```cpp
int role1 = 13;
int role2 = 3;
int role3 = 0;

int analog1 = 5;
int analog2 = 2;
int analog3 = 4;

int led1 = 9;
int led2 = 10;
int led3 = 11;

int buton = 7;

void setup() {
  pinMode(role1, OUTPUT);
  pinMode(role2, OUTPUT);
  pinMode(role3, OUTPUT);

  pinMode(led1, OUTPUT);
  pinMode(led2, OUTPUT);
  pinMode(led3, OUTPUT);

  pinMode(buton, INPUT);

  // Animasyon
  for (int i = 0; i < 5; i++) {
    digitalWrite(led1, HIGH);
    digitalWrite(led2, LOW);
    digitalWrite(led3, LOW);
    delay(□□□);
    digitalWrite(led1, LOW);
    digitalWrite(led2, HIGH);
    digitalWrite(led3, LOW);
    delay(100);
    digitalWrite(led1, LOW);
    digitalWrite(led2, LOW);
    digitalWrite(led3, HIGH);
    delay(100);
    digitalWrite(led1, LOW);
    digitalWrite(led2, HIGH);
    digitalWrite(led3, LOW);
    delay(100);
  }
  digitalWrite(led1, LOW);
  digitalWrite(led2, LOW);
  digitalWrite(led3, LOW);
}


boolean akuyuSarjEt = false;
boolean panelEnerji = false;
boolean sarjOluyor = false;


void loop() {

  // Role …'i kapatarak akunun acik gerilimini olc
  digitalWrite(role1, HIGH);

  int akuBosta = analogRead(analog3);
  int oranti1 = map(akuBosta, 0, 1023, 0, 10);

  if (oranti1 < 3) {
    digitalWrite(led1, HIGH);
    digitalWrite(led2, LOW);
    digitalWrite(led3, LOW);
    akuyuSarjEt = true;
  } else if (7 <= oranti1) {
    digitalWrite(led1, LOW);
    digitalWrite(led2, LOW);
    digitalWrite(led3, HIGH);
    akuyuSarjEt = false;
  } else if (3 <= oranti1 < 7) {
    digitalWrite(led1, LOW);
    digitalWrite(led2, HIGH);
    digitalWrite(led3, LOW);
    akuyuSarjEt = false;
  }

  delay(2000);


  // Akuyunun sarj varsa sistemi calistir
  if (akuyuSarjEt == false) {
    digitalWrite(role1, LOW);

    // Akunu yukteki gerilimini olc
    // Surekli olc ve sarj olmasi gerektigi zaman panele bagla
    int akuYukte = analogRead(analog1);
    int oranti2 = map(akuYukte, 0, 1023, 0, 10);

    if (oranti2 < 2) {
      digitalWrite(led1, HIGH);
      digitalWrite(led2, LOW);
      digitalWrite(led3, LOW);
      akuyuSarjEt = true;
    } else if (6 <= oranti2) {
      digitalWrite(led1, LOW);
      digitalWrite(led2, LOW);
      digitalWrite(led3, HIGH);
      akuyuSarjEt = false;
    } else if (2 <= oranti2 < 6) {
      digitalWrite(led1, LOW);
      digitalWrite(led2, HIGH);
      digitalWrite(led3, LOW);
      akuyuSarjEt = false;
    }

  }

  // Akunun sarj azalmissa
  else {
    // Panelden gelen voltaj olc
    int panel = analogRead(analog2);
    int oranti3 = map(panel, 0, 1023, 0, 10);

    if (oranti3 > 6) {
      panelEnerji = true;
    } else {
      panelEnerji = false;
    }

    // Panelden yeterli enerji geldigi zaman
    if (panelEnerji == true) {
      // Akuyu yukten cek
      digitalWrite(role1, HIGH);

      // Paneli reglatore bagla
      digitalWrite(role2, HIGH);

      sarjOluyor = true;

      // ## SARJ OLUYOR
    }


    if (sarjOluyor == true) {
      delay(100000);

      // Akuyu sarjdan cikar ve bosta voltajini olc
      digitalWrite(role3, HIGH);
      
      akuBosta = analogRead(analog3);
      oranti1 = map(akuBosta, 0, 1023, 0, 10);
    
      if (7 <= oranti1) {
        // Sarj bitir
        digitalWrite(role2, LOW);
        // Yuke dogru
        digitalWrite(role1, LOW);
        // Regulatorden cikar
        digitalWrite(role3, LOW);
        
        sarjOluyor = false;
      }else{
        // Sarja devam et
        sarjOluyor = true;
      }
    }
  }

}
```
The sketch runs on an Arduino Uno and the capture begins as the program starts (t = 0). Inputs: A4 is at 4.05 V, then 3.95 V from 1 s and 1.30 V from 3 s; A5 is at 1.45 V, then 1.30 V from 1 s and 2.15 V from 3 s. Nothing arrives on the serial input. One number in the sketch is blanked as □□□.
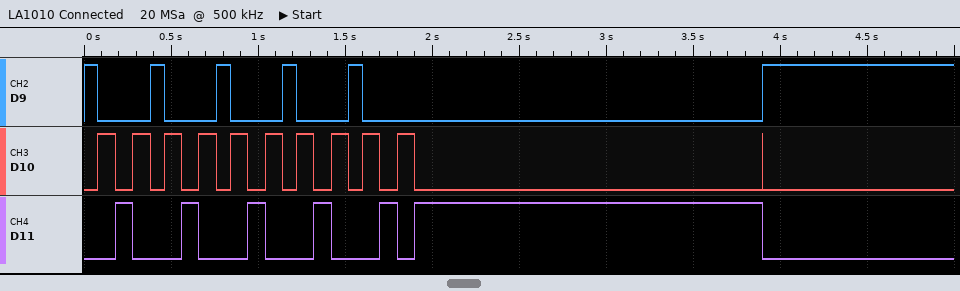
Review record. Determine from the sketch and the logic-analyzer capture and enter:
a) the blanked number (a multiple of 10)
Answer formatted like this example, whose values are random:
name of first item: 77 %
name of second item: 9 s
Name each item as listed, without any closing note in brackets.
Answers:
the blanked number: 80
